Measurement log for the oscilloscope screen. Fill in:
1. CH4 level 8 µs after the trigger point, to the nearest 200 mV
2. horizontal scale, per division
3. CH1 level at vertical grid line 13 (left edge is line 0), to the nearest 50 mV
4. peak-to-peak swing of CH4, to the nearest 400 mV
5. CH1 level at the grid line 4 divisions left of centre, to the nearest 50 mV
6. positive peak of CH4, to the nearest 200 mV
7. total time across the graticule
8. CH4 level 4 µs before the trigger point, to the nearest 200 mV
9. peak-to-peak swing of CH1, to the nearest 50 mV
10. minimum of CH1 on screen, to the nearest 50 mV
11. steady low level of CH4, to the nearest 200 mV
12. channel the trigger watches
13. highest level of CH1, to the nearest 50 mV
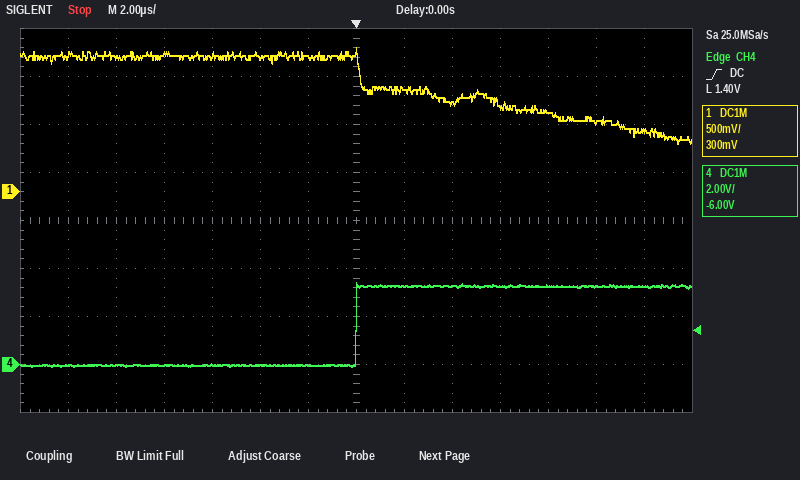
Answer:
3.2 V
2 µs
650 mV
3.6 V
1.45 V
3.4 V
28 µs
0.0 V
1.00 V
500 mV
0.0 V
CH4
1.50 V
